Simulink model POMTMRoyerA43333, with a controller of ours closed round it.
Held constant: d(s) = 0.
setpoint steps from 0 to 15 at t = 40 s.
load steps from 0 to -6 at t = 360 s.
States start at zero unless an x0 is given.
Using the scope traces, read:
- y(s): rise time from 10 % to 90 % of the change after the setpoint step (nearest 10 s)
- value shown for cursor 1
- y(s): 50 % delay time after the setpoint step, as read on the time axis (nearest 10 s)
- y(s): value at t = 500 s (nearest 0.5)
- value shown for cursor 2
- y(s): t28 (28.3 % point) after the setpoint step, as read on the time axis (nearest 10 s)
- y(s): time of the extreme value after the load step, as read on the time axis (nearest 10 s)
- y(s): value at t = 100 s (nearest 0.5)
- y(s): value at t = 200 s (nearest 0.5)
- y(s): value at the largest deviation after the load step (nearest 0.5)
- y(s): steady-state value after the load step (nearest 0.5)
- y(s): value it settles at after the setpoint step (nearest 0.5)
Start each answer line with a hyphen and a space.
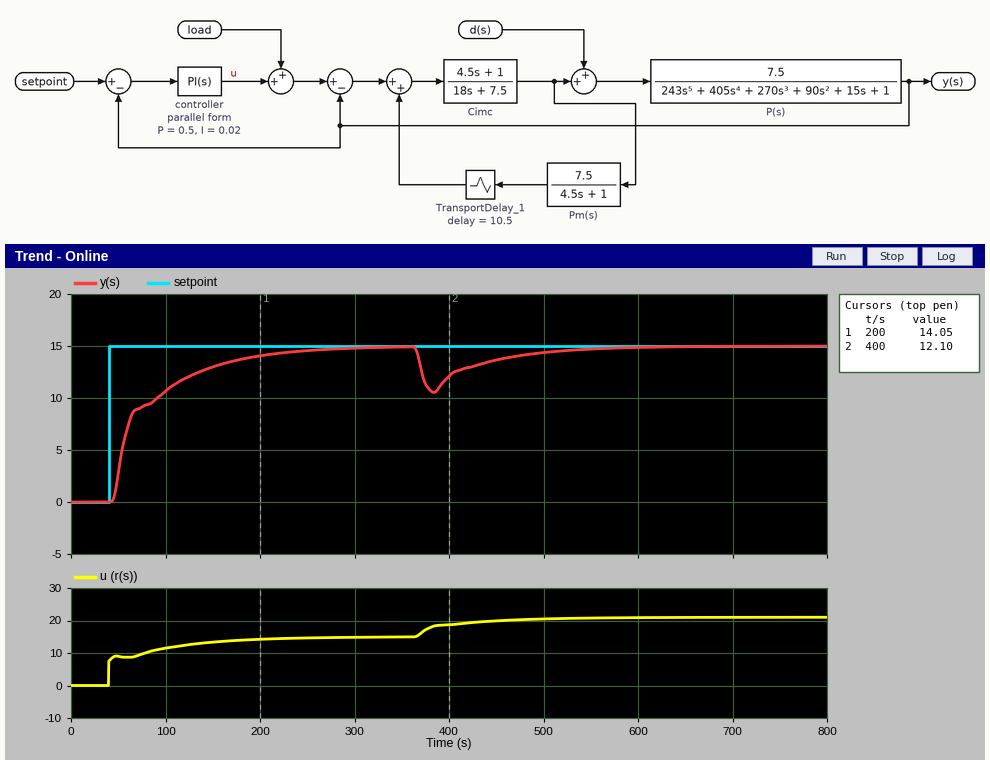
- 120 s
- 14.05
- 60 s
- 14.5
- 12.10
- 50 s
- 380 s
- 10.5
- 14.0
- 10.5
- 15.0
- 15.0
